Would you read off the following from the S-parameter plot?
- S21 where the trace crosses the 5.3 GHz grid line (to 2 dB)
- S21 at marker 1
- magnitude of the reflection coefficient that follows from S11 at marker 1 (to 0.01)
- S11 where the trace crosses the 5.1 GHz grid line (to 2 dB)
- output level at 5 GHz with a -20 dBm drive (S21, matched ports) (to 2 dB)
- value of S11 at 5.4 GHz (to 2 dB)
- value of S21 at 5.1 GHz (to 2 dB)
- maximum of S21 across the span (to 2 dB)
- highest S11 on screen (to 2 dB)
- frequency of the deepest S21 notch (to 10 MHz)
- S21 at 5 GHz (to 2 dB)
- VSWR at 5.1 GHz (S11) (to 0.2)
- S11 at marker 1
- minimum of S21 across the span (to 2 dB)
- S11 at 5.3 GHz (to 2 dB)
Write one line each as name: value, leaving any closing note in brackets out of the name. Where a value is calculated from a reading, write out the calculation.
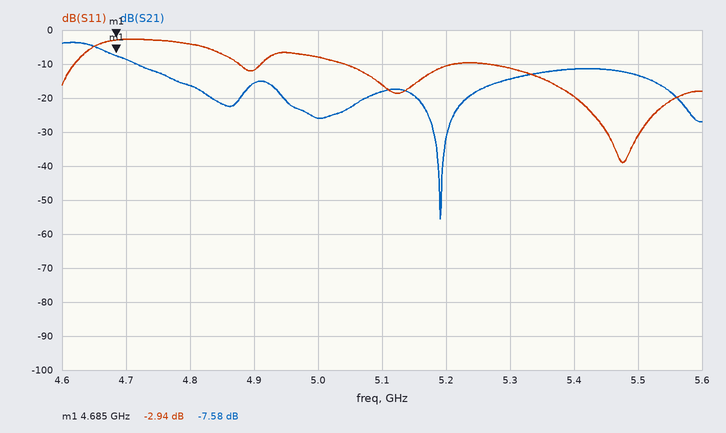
S21 where the trace crosses the 5.3 GHz grid line: -14 dB
S21 at marker 1: -7.58 dB
magnitude of the reflection coefficient that follows from S11 at marker 1: 10^(-2.94/20) ≈ 0.71
S11 where the trace crosses the 5.1 GHz grid line: -16 dB
output level at 5 GHz with a -20 dBm drive (S21, matched ports): -20 dBm + (-26 dB) = -46 dBm
value of S11 at 5.4 GHz: -20 dB
value of S21 at 5.1 GHz: -18 dB
maximum of S21 across the span: -4 dB
highest S11 on screen: -2 dB
frequency of the deepest S21 notch: 5.19 GHz
S21 at 5 GHz: -26 dB
VSWR at 5.1 GHz (S11): |Γ| = 10^(-16/20) = 0.1585; VSWR = (1 + 0.1585)/(1 − 0.1585) ≈ 1.4
S11 at marker 1: -2.94 dB
minimum of S21 across the span: -56 dB
S11 at 5.3 GHz: -12 dB
